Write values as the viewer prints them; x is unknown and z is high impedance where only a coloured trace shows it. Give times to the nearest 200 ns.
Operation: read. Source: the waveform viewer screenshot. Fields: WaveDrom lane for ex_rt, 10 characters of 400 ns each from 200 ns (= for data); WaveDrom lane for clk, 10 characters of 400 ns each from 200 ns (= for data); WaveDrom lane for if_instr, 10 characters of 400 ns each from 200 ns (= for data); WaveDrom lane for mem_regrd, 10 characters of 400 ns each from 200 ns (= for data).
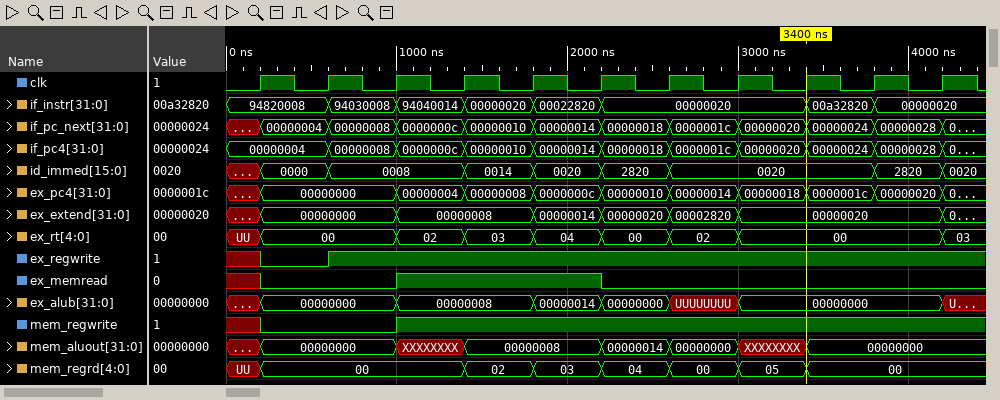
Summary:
{name: 'ex_rt', wave: '=.======..', data: '00 02 03 04 00 02 00'}
{name: 'clk', wave: 'p.........'}
{name: 'if_instr', wave: '======..==', data: '94820008 94030008 94040014 00000020 00022820 00000020 00a32820 00000020'}
{name: 'mem_regrd', wave: '=..======.', data: '00 02 03 04 00 05 00'}
